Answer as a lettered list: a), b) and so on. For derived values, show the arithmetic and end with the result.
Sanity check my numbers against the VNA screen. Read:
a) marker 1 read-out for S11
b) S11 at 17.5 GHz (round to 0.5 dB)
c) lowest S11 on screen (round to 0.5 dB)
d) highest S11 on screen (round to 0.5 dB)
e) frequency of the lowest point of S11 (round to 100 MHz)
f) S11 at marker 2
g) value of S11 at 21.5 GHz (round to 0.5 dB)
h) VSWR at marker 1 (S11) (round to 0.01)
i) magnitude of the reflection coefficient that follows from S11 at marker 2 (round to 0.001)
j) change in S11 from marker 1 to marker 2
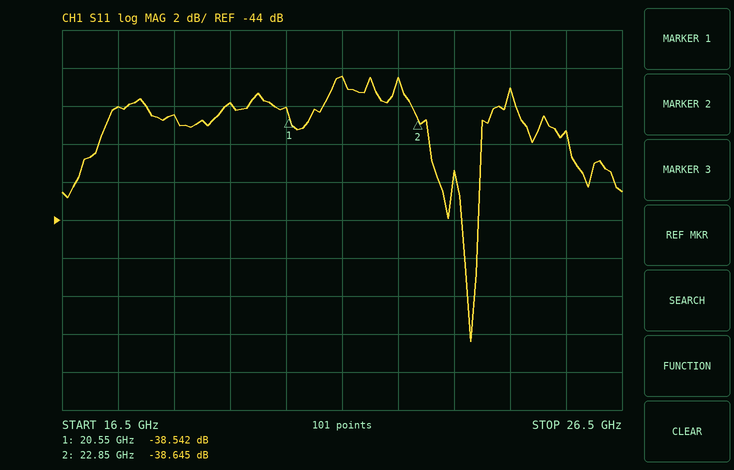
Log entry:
a) -38.542 dB
b) -38.0 dB
c) -50.5 dB
d) -36.5 dB
e) 23.8 GHz
f) -38.645 dB
g) -36.5 dB
h) (1 + 0.0118)/(1 − 0.0118) ≈ 1.02
i) 10^(-38.645/20) ≈ 0.012
j) -38.645 − (-38.542) = -0.103 dB
